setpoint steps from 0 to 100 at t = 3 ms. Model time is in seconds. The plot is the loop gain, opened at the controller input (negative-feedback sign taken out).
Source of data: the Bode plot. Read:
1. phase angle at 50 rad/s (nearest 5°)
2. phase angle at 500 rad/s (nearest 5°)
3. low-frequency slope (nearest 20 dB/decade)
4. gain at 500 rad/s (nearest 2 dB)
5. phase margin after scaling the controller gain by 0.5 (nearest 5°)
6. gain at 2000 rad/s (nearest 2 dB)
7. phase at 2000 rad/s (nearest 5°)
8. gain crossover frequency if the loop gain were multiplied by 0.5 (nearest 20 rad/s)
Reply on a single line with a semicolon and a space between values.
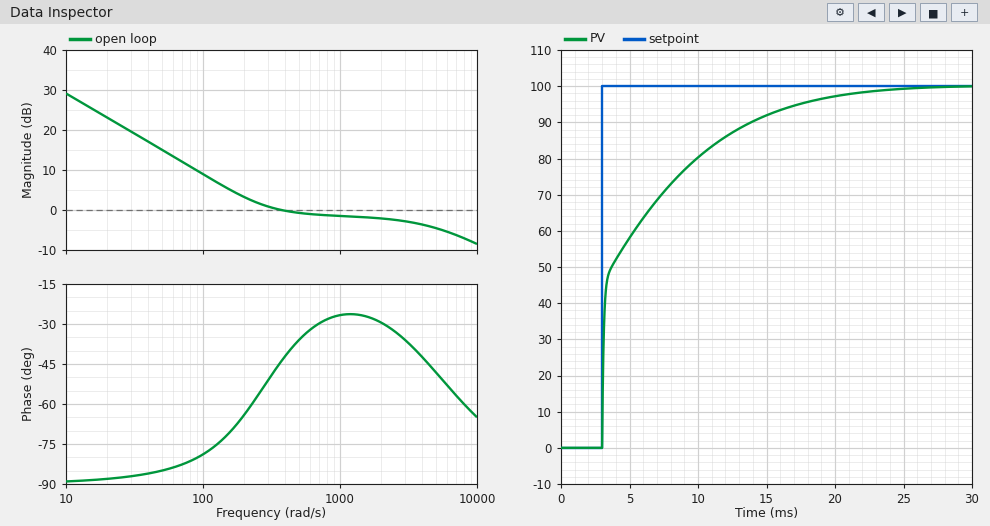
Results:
-85°; -35°; -20 dB/decade; 0 dB; 105°; -2 dB; -30°; 140 rad/s
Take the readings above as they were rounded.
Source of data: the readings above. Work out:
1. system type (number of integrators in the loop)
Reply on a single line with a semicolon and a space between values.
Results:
1
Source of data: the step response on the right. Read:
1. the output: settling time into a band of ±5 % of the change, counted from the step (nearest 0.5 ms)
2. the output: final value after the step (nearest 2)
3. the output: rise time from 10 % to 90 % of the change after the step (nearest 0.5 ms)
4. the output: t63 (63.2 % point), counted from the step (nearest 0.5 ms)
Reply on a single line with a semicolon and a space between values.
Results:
14.5 ms; 100; 11.0 ms; 3.0 ms
